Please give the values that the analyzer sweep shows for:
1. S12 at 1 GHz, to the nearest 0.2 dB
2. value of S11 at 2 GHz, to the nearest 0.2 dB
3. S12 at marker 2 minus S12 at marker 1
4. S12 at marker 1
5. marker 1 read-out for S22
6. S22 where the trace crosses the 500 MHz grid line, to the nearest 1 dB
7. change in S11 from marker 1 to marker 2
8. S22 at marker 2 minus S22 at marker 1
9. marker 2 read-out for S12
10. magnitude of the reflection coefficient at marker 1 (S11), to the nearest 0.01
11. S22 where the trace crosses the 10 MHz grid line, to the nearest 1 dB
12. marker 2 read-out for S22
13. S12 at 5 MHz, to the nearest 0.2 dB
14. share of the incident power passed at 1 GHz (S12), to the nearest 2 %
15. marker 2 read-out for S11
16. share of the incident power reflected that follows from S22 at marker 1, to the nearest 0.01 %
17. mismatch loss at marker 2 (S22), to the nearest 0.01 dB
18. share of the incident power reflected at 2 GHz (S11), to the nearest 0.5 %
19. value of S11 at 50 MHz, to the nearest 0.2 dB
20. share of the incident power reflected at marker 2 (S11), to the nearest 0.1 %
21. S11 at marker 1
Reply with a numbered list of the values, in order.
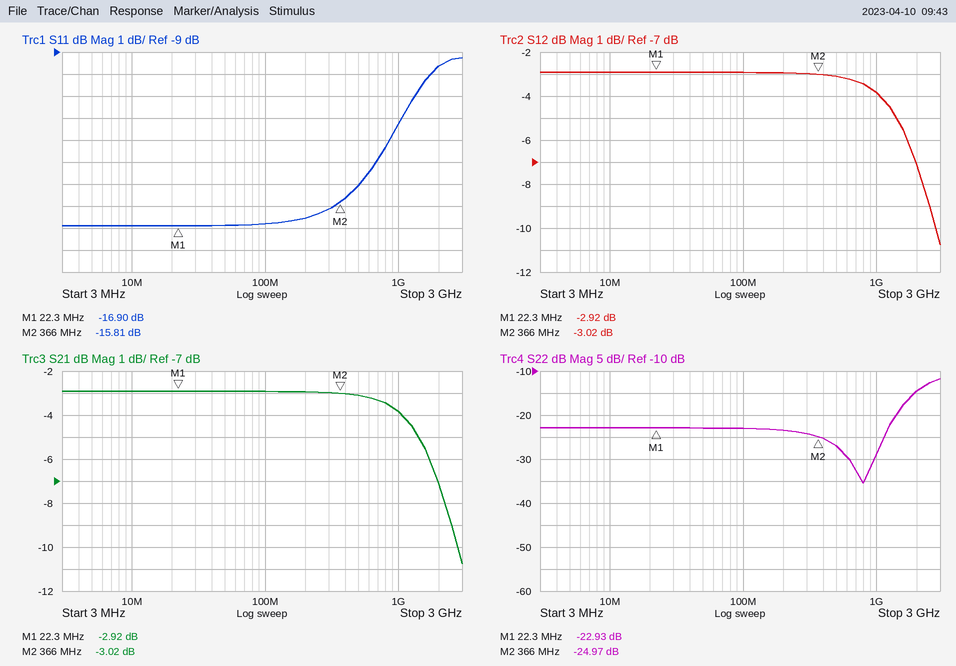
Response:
1. -3.8 dB
2. -9.6 dB
3. -0.10 dB
4. -2.92 dB
5. -22.93 dB
6. -27 dB
7. 1.09 dB
8. -2.04 dB
9. -3.02 dB
10. 0.14
11. -23 dB
12. -24.97 dB
13. -3.0 dB
14. 42 %
15. -15.81 dB
16. 0.51 %
17. 0.01 dB
18. 11.0 %
19. -16.8 dB
20. 2.6 %
21. -16.90 dB
